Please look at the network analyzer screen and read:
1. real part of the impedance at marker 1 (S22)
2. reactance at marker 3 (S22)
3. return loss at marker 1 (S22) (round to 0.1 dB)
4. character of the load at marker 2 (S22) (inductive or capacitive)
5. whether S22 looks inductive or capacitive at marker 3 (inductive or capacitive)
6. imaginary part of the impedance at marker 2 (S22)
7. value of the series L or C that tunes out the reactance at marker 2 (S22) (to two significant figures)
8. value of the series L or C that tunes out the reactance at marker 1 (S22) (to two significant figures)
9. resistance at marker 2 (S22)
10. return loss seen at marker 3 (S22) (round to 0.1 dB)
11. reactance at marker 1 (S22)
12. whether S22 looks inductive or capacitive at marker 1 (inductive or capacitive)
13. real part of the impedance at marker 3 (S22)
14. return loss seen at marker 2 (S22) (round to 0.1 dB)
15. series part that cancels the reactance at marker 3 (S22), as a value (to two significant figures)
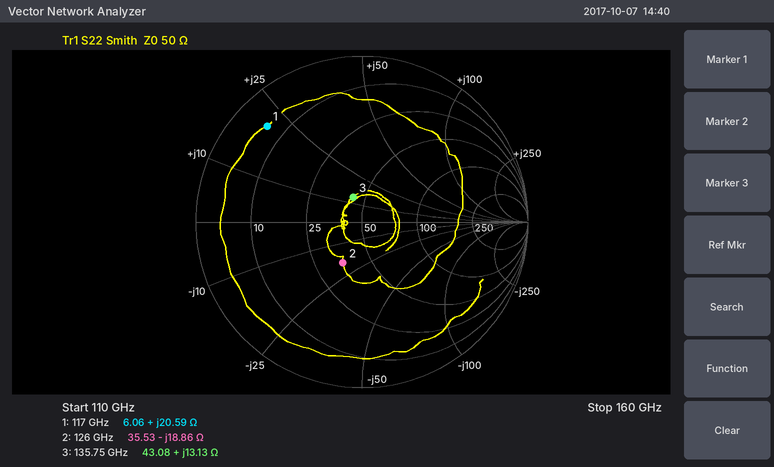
6.06 Ω
+13.13 Ω
1.8 dB
capacitive
inductive
-18.86 Ω
24 pH
66 fF
35.53 Ω
16.0 dB
+20.59 Ω
inductive
43.08 Ω
11.3 dB
89 fF
